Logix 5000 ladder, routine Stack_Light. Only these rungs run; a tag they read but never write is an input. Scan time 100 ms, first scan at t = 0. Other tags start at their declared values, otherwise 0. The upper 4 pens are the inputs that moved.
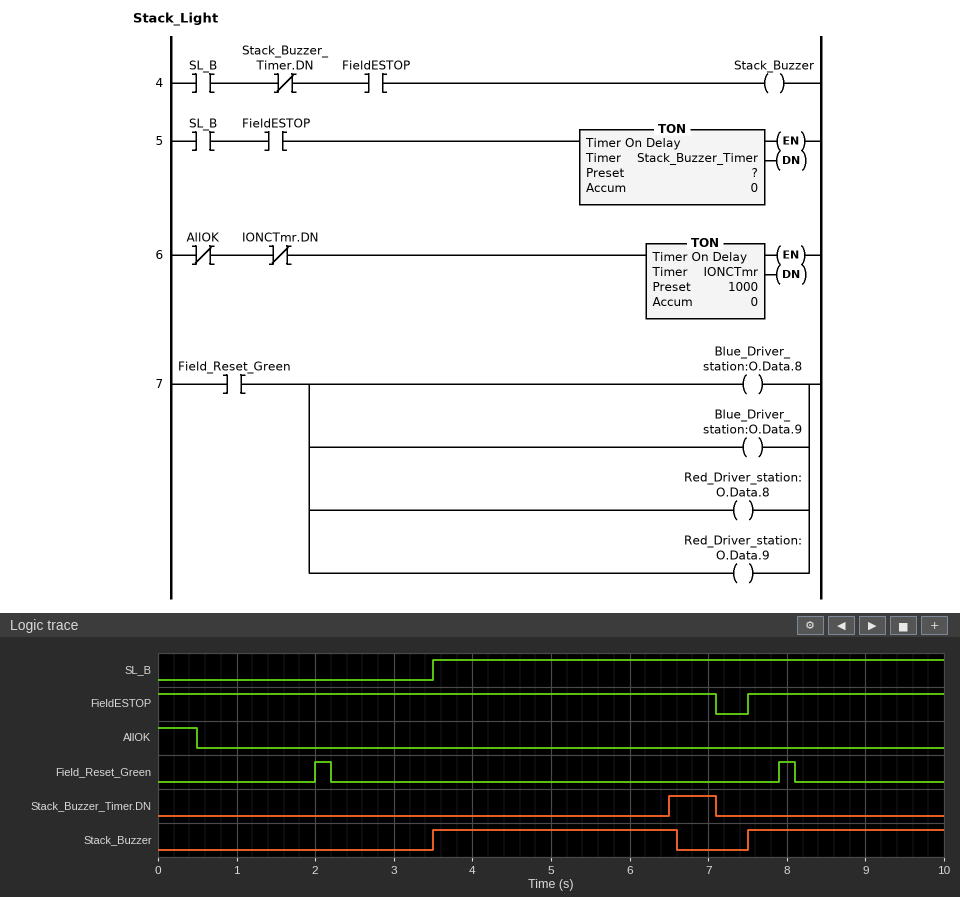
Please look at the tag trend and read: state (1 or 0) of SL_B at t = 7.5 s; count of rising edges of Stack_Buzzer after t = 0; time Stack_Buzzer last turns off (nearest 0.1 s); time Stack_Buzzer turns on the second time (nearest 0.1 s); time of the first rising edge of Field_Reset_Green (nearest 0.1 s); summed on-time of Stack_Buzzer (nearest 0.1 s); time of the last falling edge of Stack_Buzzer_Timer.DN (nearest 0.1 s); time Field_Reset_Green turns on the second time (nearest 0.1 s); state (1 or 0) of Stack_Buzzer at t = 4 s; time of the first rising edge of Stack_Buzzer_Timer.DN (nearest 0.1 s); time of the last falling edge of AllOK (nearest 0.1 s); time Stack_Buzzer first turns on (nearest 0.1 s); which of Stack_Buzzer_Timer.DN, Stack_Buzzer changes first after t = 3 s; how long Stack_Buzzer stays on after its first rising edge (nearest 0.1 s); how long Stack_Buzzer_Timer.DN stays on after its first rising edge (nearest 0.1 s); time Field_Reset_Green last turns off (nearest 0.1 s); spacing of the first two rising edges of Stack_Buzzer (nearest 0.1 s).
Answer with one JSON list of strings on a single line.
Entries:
["1", "2", "6.6 s", "7.5 s", "2.0 s", "5.6 s", "7.1 s", "7.9 s", "1", "6.5 s", "0.5 s", "3.5 s", "Stack_Buzzer", "3.1 s", "0.6 s", "8.1 s", "4.0 s"]
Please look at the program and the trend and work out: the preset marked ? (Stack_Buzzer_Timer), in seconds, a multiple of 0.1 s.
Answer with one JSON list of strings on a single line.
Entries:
["3.0 s"]
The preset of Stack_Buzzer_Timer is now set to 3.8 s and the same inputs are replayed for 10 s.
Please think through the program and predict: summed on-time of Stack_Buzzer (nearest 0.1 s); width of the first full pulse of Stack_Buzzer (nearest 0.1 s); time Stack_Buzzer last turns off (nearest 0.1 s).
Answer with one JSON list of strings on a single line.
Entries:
["6.1 s", "3.6 s", "7.1 s"]
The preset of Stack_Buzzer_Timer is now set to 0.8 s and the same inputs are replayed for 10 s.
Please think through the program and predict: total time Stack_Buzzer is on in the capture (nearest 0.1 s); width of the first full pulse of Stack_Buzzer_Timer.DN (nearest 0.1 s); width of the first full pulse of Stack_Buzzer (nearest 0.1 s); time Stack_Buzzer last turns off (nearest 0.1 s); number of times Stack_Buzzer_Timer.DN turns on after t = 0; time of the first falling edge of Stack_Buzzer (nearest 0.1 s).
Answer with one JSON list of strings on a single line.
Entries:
["1.8 s", "2.8 s", "0.9 s", "8.4 s", "2", "4.4 s"]
